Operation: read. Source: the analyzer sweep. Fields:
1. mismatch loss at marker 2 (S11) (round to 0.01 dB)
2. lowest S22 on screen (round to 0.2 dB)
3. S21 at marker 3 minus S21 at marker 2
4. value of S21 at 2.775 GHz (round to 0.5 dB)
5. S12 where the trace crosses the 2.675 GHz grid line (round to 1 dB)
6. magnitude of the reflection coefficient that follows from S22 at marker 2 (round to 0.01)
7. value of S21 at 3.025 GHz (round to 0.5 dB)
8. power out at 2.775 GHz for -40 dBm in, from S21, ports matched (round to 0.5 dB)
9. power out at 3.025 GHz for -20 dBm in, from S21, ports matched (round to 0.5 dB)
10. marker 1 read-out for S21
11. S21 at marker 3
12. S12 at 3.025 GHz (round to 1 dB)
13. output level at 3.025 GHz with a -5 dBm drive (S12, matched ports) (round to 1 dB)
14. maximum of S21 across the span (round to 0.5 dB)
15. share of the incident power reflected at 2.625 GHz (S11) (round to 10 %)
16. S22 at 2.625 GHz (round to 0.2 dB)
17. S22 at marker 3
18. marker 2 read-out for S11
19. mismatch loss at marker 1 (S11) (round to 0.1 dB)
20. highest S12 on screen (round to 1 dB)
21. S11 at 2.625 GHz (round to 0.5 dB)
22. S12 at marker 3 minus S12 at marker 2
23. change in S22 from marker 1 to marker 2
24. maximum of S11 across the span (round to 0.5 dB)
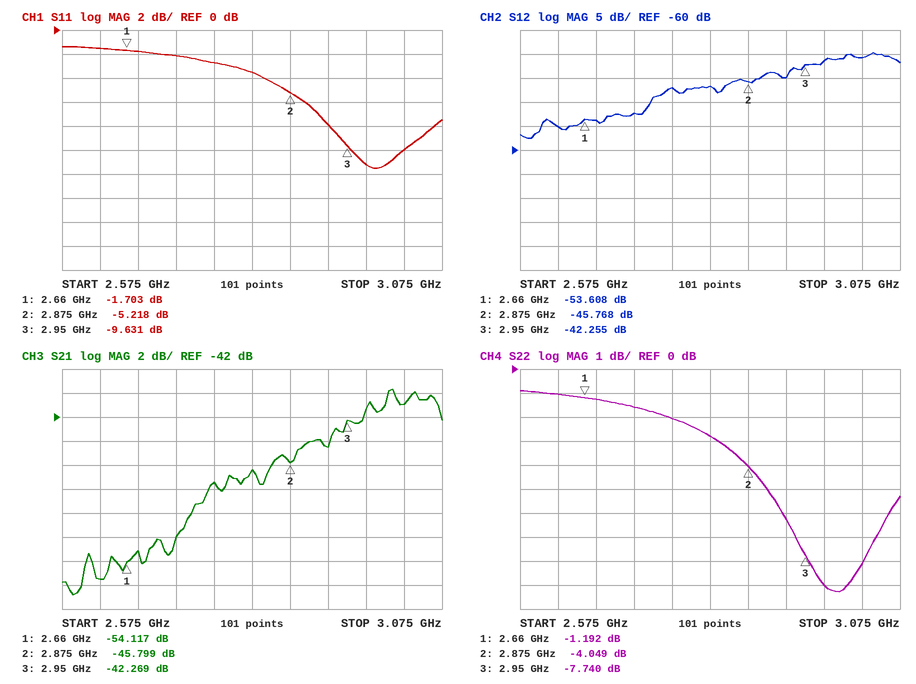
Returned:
1.55 dB
-9.2 dB
3.530 dB
-47.5 dB
-54 dB
0.63
-41.0 dB
-87.5 dBm
-61.0 dBm
-54.117 dB
-42.269 dB
-41 dB
-46 dBm
-39.5 dB
70 %
-1.0 dB
-7.740 dB
-5.218 dB
4.9 dB
-40 dB
-1.5 dB
3.513 dB
-2.857 dB
-1.5 dB
